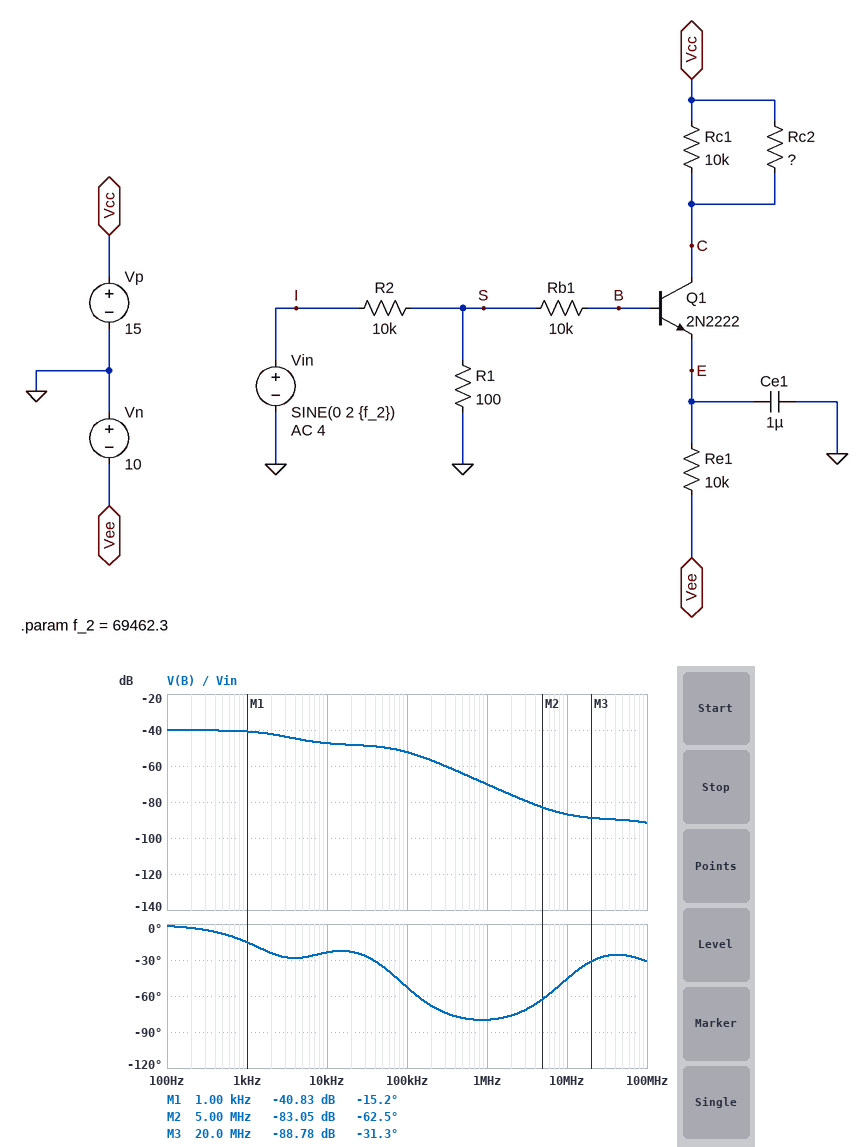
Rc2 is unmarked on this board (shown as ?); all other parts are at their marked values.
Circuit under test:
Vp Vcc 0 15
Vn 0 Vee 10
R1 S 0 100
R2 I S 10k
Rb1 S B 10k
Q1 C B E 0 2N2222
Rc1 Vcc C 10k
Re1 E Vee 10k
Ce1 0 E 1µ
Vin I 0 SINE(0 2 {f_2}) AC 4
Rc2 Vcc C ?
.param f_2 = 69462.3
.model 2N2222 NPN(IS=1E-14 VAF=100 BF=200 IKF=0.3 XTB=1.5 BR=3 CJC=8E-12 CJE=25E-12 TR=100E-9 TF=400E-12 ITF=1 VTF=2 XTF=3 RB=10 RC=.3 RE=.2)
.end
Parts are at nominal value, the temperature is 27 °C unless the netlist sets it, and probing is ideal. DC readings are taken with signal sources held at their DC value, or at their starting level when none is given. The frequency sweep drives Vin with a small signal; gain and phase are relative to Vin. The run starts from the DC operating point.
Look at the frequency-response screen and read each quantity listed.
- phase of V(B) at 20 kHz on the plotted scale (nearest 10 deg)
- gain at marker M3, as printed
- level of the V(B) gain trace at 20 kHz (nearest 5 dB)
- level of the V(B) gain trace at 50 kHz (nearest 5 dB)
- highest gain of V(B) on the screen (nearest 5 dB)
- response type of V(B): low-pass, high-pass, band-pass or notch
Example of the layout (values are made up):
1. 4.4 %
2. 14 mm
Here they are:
1. -20 deg
2. -88.78 dB
3. -50 dB
4. -50 dB
5. -40 dB
6. low-pass
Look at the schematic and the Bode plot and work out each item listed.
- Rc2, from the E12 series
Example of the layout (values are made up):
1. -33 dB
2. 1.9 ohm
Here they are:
1. 6.8 kΩ
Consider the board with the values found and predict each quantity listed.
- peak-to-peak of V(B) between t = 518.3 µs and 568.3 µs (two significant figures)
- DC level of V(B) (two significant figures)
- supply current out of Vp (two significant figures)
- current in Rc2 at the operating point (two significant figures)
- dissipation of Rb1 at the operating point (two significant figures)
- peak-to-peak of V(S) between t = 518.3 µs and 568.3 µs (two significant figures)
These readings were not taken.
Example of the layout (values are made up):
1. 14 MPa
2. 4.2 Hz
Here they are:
1. 12 mV
2. -42 mV
3. 930 µA
4. 550 µA
5. 170 nW
6. 39 mV
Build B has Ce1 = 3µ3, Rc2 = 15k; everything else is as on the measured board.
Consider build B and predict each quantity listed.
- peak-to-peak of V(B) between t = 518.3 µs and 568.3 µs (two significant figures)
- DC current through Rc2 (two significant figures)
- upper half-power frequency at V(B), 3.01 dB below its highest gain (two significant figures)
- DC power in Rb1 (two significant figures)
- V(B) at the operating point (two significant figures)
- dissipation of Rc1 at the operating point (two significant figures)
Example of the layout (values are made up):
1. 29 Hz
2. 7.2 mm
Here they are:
1. 9.5 mV
2. 370 µA
3. 750 Hz
4. 180 nW
5. -43 mV
6. 3.1 mW
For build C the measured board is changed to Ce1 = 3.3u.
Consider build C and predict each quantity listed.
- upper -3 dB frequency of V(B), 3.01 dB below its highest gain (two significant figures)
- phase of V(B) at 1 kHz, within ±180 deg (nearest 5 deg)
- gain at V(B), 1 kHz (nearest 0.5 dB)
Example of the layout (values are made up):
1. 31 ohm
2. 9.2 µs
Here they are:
1. 770 Hz
2. -25 deg
3. -44.0 dB
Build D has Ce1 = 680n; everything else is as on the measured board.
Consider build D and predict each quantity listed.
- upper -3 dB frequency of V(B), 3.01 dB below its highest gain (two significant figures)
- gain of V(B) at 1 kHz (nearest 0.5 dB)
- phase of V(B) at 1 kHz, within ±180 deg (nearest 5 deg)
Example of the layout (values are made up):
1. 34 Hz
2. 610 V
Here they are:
1. 3.9 kHz
2. -40.5 dB
3. -10 deg
